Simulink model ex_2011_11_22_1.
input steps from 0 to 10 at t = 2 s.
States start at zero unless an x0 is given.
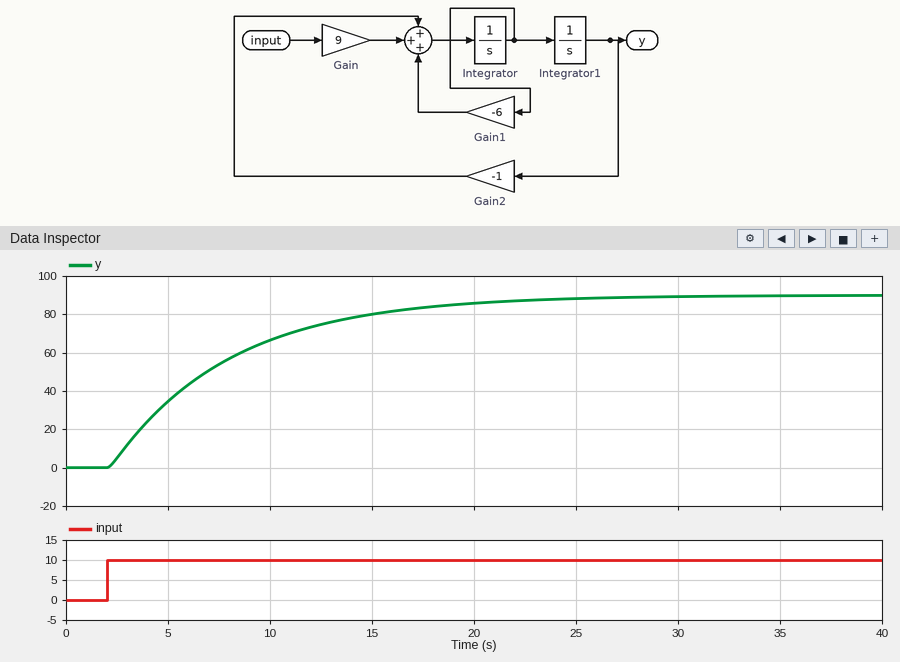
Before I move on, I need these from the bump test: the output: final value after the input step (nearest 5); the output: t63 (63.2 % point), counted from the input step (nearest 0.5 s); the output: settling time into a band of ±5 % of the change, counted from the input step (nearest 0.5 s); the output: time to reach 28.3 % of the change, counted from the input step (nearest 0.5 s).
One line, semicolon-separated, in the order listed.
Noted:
90; 6.0 s; 17.5 s; 2.0 s
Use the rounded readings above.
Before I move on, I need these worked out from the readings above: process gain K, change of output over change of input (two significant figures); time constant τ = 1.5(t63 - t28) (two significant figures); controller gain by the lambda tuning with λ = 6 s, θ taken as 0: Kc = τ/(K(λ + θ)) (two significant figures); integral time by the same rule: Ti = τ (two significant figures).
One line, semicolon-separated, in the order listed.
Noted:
9.0; 6.0 s; 0.11; 6.0 s
